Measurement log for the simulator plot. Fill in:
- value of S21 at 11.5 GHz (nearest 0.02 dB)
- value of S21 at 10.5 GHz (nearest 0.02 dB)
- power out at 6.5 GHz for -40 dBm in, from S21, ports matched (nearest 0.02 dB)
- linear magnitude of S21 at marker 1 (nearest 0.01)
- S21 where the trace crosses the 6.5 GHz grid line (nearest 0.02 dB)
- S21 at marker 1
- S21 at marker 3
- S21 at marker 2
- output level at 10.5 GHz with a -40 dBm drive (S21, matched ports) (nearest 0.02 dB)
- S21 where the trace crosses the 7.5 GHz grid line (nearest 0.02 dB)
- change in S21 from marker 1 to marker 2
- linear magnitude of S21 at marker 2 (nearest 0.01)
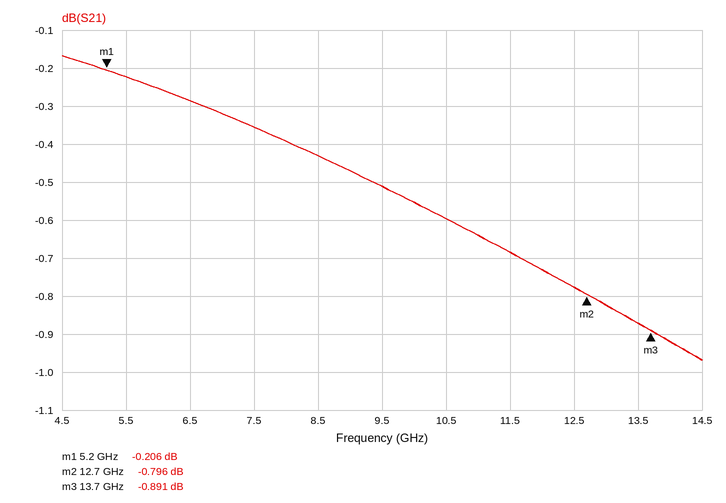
-0.68 dB
-0.60 dB
-40.28 dBm
0.98
-0.28 dB
-0.206 dB
-0.891 dB
-0.796 dB
-40.60 dBm
-0.36 dB
-0.590 dB
0.91
